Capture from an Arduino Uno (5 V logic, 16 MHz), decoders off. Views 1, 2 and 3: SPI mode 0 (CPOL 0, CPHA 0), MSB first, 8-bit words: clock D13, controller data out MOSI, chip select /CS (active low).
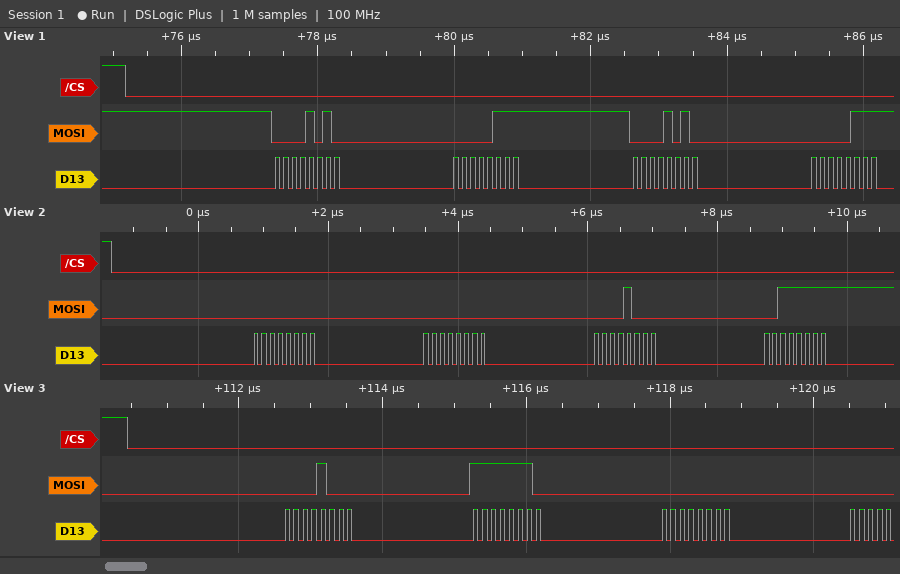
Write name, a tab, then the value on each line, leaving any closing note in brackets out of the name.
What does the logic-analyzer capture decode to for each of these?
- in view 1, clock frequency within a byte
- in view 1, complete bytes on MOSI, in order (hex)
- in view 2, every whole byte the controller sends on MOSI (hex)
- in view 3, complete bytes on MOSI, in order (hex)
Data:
in view 1, clock frequency within a byte	8 MHz
in view 1, complete bytes on MOSI, in order	0A 07 0A 07
in view 2, every whole byte the controller sends on MOSI	00 00 08 3F
in view 3, complete bytes on MOSI, in order	08 FE 00
